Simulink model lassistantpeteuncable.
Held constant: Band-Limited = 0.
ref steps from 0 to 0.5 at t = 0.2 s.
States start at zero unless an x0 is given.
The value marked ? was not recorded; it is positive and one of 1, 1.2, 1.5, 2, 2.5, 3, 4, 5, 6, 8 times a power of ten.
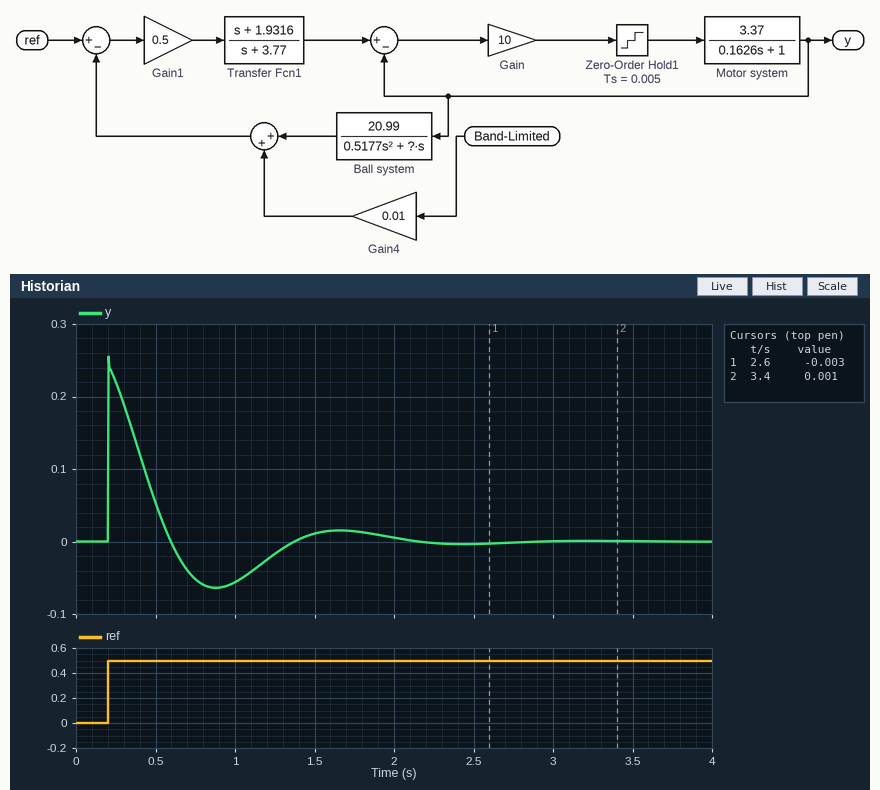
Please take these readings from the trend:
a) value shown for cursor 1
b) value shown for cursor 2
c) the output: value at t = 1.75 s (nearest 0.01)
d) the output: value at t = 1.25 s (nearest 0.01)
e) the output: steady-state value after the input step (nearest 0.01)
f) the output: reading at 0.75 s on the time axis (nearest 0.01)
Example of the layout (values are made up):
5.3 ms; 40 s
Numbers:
-0.003; 0.001; 0.01; -0.02; 0.00; -0.05
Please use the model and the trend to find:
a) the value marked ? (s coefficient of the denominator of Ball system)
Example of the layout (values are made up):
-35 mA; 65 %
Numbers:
1
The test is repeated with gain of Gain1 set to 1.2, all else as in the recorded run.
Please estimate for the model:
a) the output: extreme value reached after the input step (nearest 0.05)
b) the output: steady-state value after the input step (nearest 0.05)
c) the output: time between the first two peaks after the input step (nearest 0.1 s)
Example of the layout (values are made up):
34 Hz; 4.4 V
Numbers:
0.60; 0.00; 0.9 s
